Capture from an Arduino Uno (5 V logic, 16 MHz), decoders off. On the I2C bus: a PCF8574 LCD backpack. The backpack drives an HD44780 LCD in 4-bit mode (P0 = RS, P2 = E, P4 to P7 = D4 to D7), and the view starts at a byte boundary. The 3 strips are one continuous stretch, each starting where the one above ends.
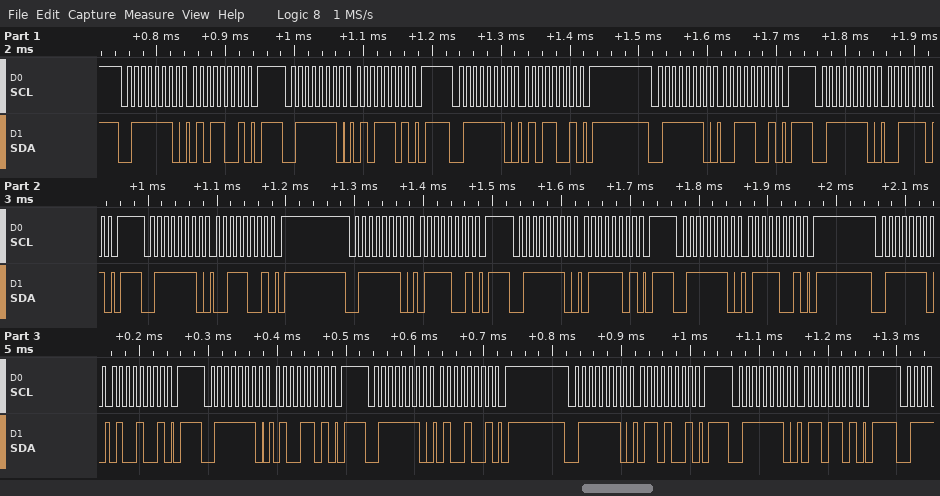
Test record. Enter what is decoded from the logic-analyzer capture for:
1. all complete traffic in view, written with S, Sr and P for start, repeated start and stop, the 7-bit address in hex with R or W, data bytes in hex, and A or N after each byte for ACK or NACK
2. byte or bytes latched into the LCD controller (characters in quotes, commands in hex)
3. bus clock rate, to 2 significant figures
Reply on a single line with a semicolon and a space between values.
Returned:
S 3FW A 59 A P S 3FW A 5D A P S 3FW A 59 A P S 3FW A 39 A P S 3FW A 3D A P S 3FW A 39 A P S 3FW A 79 A P S 3FW A 7D A P S 3FW A 79 A P S 3FW A 49 A P S 3FW A 4D A P S 3FW A 49 A P S 3FW A 69 A P S 3FW A 6D A P; 'S' 't'; 100 kHz
